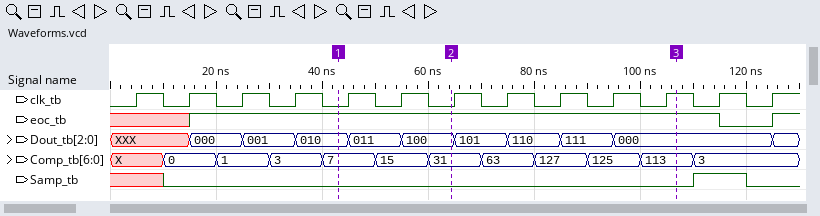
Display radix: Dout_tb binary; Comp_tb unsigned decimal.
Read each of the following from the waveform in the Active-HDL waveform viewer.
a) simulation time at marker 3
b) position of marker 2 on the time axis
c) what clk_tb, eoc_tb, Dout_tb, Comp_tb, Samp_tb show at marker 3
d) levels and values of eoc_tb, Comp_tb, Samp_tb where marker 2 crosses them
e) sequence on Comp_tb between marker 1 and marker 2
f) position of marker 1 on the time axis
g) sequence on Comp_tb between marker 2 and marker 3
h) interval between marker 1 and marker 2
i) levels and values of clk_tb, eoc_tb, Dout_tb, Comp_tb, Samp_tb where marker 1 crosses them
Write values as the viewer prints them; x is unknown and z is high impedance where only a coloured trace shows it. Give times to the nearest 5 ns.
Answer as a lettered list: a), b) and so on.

a) 105 ns
b) 65 ns
c) clk_tb=1, eoc_tb=1, Dout_tb=000, Comp_tb=113, Samp_tb=0
d) eoc_tb=1, Comp_tb=31, Samp_tb=0
e) 7, 15, 31
f) 45 ns
g) 31, 63, 127, 125, 113
h) 20 ns
i) clk_tb=0, eoc_tb=1, Dout_tb=010, Comp_tb=7, Samp_tb=0
